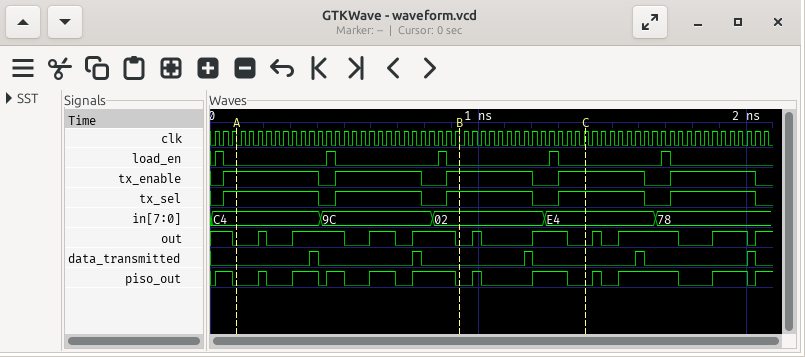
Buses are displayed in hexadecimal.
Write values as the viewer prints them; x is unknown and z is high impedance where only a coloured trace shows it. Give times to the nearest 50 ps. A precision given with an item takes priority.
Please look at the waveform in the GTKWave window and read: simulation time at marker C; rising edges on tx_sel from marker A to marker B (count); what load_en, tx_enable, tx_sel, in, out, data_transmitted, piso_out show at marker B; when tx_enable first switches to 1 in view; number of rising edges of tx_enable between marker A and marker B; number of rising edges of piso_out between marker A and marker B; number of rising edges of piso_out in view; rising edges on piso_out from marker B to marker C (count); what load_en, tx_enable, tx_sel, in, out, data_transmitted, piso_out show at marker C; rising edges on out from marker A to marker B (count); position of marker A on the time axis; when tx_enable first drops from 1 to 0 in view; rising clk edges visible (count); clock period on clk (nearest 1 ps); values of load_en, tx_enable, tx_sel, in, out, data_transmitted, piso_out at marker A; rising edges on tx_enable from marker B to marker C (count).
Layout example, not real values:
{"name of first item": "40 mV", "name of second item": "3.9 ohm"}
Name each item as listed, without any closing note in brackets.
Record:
{"simulation time at marker C": "1400 ps", "rising edges on tx_sel from marker A to marker B": "2", "what load_en, tx_enable, tx_sel, in, out, data_transmitted, piso_out show at marker B": "load_en=0, tx_enable=1, tx_sel=1, in=02, out=0, data_transmitted=0, piso_out=0", "when tx_enable first switches to 1 in view": "50 ps", "number of rising edges of tx_enable between marker A and marker B": "2", "number of rising edges of piso_out between marker A and marker B": "5", "number of rising edges of piso_out in view": "12", "rising edges on piso_out from marker B to marker C": "2", "what load_en, tx_enable, tx_sel, in, out, data_transmitted, piso_out show at marker C": "load_en=0, tx_enable=1, tx_sel=1, in=E4, out=0, data_transmitted=0, piso_out=0", "rising edges on out from marker A to marker B": "4", "position of marker A on the time axis": "100 ps", "when tx_enable first drops from 1 to 0 in view": "400 ps", "rising clk edges visible": "65", "clock period on clk": "32 ps", "values of load_en, tx_enable, tx_sel, in, out, data_transmitted, piso_out at marker A": "load_en=0, tx_enable=1, tx_sel=1, in=C4, out=0, data_transmitted=0, piso_out=0", "rising edges on tx_enable from marker B to marker C": "1"}
